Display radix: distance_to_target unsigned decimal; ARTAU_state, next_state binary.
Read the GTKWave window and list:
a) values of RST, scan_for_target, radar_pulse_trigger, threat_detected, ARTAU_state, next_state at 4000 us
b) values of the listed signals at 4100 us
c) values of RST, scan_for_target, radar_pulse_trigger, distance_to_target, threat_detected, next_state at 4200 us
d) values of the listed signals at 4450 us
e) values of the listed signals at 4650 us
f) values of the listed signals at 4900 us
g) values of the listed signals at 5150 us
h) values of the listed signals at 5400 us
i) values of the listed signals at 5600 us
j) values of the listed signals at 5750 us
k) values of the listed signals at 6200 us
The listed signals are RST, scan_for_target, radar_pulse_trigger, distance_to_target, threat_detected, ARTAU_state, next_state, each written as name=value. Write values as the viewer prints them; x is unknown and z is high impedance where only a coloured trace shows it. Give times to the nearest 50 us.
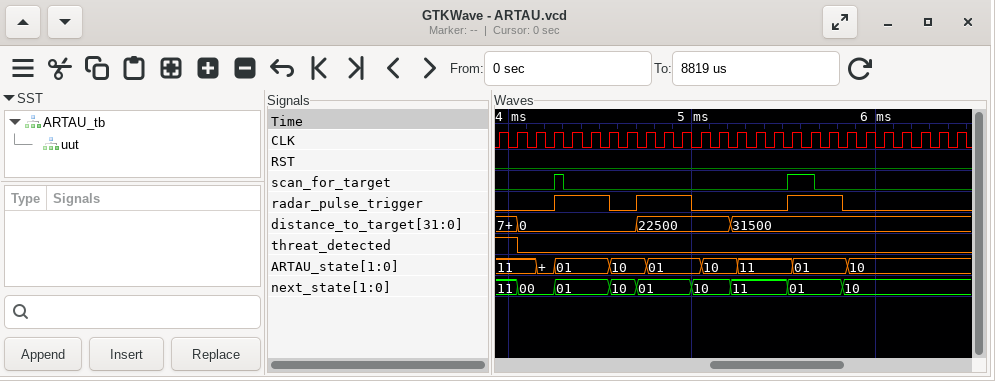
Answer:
RST=0, scan_for_target=0, radar_pulse_trigger=0, threat_detected=1, ARTAU_state=11, next_state=11
RST=0, scan_for_target=0, radar_pulse_trigger=0, distance_to_target=0, threat_detected=0, ARTAU_state=11, next_state=00
RST=0, scan_for_target=0, radar_pulse_trigger=0, distance_to_target=0, threat_detected=0, next_state=00
RST=0, scan_for_target=0, radar_pulse_trigger=1, distance_to_target=0, threat_detected=0, ARTAU_state=01, next_state=01
RST=0, scan_for_target=0, radar_pulse_trigger=0, distance_to_target=0, threat_detected=0, ARTAU_state=10, next_state=10
RST=0, scan_for_target=0, radar_pulse_trigger=1, distance_to_target=22500, threat_detected=0, ARTAU_state=01, next_state=01
RST=0, scan_for_target=0, radar_pulse_trigger=0, distance_to_target=22500, threat_detected=0, ARTAU_state=10, next_state=10
RST=0, scan_for_target=0, radar_pulse_trigger=0, distance_to_target=31500, threat_detected=0, ARTAU_state=11, next_state=11
RST=0, scan_for_target=1, radar_pulse_trigger=1, distance_to_target=31500, threat_detected=0, ARTAU_state=01, next_state=01
RST=0, scan_for_target=0, radar_pulse_trigger=1, distance_to_target=31500, threat_detected=0, ARTAU_state=01, next_state=01
RST=0, scan_for_target=0, radar_pulse_trigger=0, distance_to_target=31500, threat_detected=0, ARTAU_state=10, next_state=10
